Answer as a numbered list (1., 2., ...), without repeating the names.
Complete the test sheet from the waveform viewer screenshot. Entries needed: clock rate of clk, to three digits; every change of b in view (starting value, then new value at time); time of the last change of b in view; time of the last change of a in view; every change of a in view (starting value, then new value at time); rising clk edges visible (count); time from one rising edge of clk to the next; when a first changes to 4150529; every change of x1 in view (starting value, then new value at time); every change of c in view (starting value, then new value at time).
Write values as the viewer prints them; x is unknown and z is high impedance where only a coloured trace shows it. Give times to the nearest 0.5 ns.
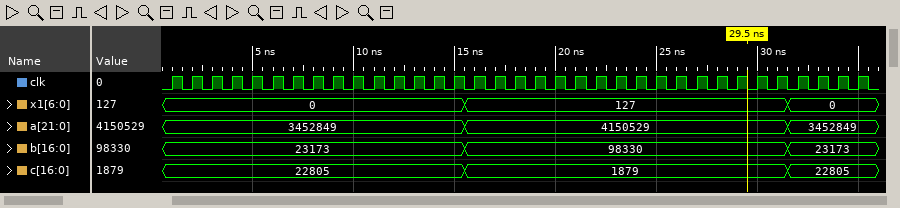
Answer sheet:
1. 1.00 GHz
2. 23173, 98330 at 15.5 ns, 23173 at 31.5 ns
3. 31.5 ns
4. 31.5 ns
5. 3452849, 4150529 at 15.5 ns, 3452849 at 31.5 ns
6. 35
7. 1 ns
8. 15.5 ns
9. 0, 127 at 15.5 ns, 0 at 31.5 ns
10. 22805, 1879 at 15.5 ns, 22805 at 31.5 ns
